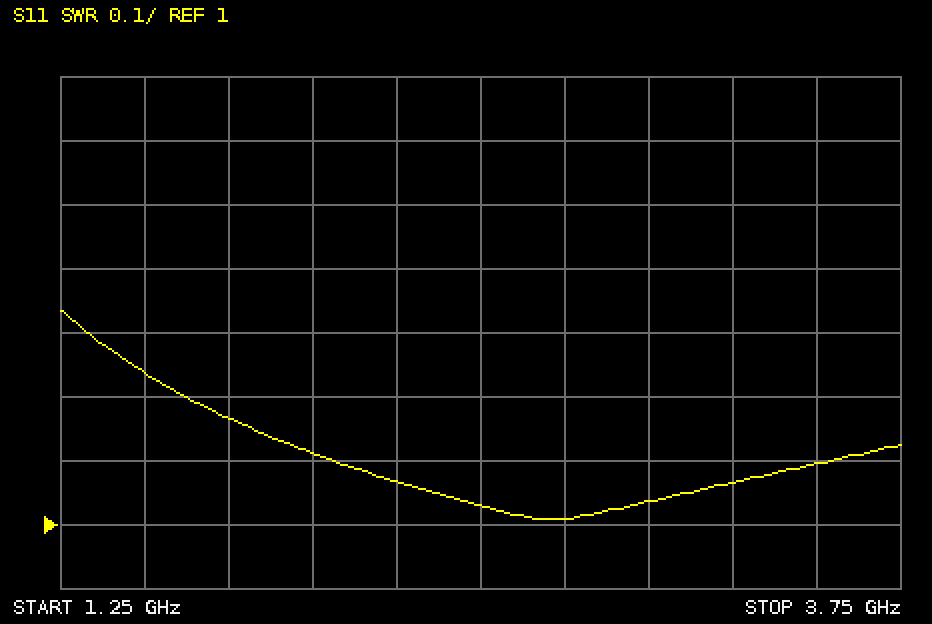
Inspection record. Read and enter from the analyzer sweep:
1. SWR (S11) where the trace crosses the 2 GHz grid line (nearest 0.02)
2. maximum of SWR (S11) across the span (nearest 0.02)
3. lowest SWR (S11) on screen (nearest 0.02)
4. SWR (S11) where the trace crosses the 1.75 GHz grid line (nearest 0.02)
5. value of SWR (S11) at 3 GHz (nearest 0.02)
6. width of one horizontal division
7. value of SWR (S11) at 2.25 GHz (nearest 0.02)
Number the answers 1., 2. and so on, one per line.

1. 1.12
2. 1.34
3. 1.00
4. 1.16
5. 1.04
6. 250 MHz
7. 1.06
